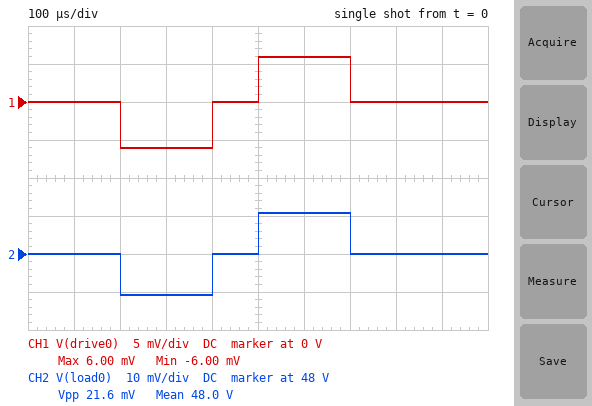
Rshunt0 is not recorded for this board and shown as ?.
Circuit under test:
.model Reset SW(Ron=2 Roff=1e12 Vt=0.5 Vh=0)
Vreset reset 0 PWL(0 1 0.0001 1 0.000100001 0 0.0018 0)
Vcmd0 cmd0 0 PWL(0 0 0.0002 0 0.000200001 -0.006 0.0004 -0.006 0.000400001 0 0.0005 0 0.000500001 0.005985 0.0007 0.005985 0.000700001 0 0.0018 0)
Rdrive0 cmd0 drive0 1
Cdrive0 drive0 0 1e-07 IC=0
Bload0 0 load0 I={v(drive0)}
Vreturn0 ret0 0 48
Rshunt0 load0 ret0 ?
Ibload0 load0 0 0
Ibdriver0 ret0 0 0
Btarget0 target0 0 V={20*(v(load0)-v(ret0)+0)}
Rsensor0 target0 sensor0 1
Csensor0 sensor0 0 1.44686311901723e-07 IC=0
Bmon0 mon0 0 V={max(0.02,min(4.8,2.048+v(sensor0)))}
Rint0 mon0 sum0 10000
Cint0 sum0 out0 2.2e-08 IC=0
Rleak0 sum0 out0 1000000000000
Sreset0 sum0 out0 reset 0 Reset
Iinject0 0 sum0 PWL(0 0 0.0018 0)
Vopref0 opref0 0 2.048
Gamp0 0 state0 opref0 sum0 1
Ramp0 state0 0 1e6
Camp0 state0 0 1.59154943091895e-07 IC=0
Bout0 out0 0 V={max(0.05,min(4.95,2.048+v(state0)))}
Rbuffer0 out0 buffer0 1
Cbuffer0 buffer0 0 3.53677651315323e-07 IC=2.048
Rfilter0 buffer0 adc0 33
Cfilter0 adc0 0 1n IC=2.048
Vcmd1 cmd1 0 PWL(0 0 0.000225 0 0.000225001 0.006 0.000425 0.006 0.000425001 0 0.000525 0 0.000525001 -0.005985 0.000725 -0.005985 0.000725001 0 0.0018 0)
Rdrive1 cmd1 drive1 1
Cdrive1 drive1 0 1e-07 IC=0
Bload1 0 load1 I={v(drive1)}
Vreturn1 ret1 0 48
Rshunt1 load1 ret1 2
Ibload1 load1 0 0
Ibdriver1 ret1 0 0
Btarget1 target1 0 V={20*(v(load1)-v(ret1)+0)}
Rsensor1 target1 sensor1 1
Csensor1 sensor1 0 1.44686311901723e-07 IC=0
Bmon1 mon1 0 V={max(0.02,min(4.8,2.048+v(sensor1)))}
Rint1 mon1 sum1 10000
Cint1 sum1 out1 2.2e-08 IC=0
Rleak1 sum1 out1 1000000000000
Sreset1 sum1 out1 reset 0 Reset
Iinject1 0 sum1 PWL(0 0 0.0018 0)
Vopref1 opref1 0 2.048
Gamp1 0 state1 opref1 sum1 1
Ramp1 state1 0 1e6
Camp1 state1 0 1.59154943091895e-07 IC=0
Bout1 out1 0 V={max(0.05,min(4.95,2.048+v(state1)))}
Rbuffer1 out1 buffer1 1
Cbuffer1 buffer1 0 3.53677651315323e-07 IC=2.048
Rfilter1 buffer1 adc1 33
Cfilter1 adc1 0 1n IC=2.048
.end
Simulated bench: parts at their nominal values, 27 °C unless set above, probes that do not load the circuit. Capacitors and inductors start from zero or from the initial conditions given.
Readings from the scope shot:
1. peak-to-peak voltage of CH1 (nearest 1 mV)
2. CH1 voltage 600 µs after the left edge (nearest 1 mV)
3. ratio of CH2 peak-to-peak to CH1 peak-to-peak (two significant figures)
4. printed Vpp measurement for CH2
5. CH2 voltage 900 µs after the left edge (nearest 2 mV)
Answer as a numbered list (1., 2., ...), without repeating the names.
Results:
1. 12 mV
2. 6 mV
3. 1.8
4. 21.6 mV
5. 48.000 V
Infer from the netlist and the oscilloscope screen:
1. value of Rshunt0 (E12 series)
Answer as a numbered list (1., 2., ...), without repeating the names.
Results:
1. 1.8 Ω
